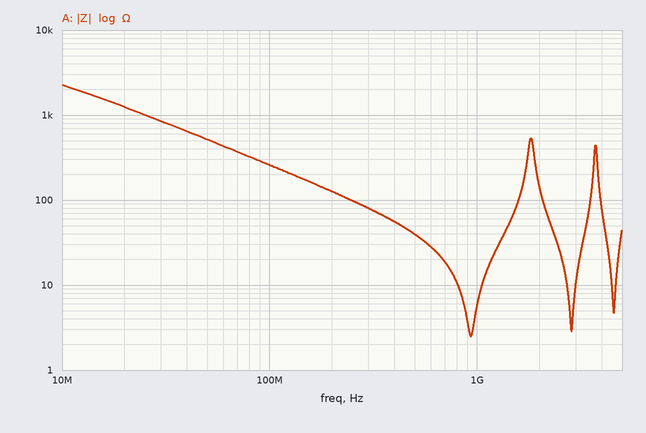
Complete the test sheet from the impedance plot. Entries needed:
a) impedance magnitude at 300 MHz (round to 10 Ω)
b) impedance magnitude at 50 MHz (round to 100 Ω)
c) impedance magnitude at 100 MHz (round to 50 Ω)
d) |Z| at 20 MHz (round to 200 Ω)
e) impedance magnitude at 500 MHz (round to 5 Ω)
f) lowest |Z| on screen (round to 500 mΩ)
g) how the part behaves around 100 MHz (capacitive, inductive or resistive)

80 Ω
500 Ω
250 Ω
1.2 kΩ
40 Ω
2.5 Ω
capacitive
